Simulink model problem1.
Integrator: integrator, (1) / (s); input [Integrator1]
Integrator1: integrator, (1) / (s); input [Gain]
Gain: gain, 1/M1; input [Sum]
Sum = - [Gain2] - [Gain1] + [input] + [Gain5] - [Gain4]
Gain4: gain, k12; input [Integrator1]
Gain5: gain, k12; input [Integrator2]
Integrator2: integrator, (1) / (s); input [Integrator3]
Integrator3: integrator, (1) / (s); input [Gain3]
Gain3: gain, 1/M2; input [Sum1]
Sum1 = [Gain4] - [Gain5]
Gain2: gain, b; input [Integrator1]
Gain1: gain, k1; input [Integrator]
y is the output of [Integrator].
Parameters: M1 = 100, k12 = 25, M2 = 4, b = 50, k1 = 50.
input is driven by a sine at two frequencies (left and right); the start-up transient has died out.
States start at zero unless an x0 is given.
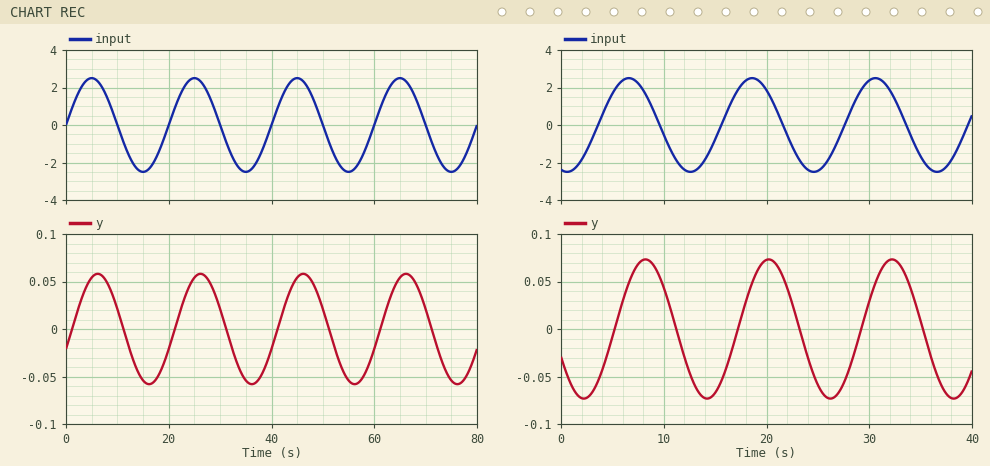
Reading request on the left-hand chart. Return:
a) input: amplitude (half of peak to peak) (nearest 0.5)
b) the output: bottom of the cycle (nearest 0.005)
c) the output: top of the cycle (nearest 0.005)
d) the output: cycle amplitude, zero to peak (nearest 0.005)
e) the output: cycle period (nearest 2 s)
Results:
2.5
-0.060
0.060
0.060
20 s
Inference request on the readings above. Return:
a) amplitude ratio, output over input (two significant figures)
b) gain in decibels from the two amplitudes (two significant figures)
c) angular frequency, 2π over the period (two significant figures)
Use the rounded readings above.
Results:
0.024
-32 dB
0.31 rad/s
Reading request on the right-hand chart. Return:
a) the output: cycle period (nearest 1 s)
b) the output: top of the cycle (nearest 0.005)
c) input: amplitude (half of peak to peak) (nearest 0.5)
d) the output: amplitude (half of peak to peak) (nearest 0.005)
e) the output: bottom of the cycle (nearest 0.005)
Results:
12 s
0.075
2.5
0.075
-0.075
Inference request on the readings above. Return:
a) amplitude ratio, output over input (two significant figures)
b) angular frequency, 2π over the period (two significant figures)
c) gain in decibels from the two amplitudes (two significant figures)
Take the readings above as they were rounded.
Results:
0.030
0.52 rad/s
-30 dB
